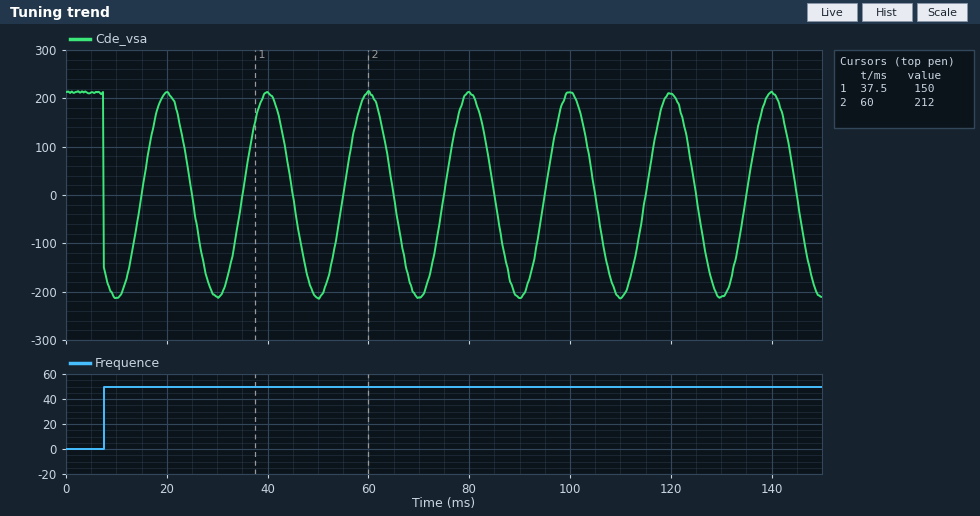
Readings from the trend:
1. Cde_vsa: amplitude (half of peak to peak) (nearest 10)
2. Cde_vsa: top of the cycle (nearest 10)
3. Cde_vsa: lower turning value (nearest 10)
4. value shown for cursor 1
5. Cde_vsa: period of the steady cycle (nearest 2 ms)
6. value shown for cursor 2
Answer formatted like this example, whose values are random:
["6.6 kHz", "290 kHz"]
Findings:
["210", "210", "-210", "150", "20 ms", "212"]
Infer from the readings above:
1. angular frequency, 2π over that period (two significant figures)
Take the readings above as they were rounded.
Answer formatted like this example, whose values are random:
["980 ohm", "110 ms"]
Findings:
["0.31 rad/ms"]
